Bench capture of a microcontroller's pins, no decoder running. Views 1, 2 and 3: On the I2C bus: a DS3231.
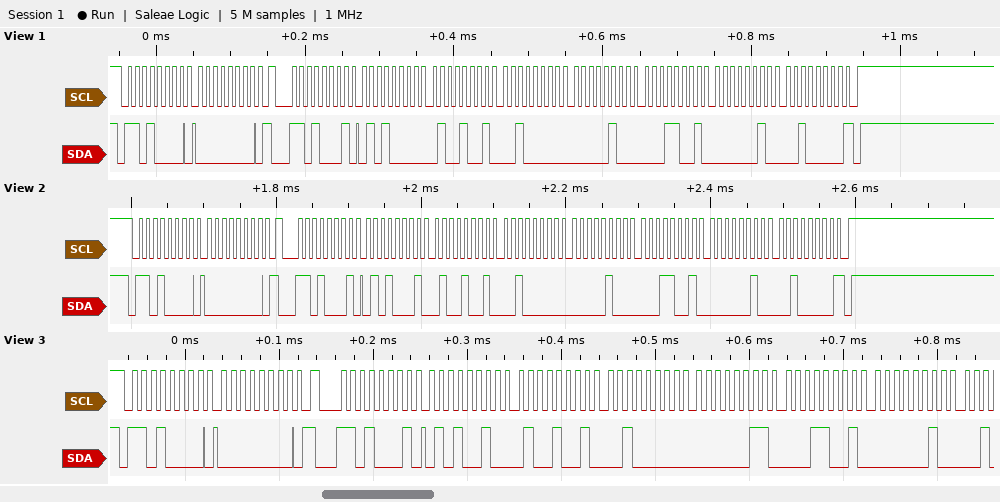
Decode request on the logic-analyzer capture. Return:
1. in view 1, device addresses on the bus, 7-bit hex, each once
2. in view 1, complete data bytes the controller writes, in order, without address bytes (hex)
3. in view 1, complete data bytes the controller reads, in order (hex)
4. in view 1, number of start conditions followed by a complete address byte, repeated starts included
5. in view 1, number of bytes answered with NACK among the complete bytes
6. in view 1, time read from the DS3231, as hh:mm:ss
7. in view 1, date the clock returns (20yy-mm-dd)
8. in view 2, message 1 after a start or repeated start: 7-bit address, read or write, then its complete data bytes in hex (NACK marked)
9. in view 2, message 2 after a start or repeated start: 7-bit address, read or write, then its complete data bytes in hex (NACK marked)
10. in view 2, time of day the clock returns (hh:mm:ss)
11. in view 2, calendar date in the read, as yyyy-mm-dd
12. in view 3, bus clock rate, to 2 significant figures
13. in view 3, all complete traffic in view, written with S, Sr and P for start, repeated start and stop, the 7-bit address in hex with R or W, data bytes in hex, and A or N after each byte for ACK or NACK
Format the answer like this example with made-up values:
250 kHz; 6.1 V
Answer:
0x68; 00; 50 49 20 04 19 02 20; 2; 1; 20:49:50; 2020-02-19; 0x68 write: 00; 0x68 read: 51 49 20 04 19 02 20 NACK; 20:49:51; 2020-02-19; 100 kHz; S 68W A 00 A Sr 68R A 52 A 49 A 20 A 03 A 19 A 02 A
